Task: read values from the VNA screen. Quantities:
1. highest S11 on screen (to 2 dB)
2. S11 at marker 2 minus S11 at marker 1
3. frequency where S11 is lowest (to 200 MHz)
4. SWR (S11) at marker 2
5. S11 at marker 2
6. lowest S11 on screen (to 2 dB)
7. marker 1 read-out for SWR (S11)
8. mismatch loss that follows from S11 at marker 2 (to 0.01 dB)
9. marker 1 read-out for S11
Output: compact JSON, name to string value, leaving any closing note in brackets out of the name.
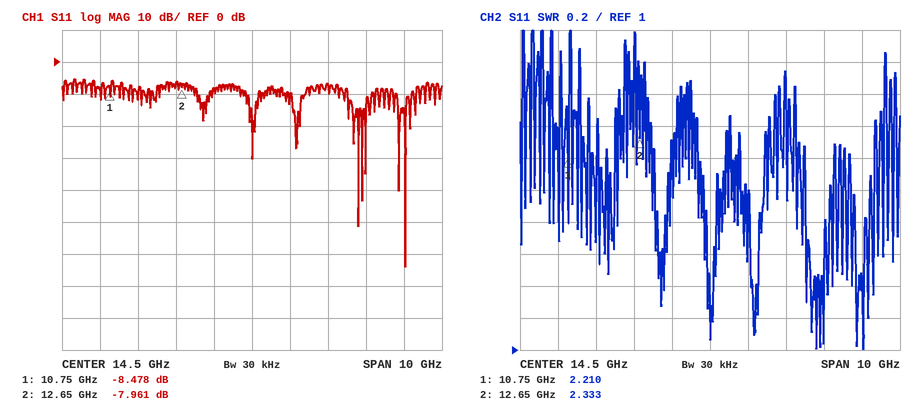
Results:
{"highest S11 on screen": "-6 dB", "S11 at marker 2 minus S11 at marker 1": "0.517 dB", "frequency where S11 is lowest": "18.6 GHz", "SWR (S11) at marker 2": "2.333", "S11 at marker 2": "-7.961 dB", "lowest S11 on screen": "-64 dB", "marker 1 read-out for SWR": "2.210", "mismatch loss that follows from S11 at marker 2": "0.76 dB", "marker 1 read-out for S11": "-8.478 dB"}
